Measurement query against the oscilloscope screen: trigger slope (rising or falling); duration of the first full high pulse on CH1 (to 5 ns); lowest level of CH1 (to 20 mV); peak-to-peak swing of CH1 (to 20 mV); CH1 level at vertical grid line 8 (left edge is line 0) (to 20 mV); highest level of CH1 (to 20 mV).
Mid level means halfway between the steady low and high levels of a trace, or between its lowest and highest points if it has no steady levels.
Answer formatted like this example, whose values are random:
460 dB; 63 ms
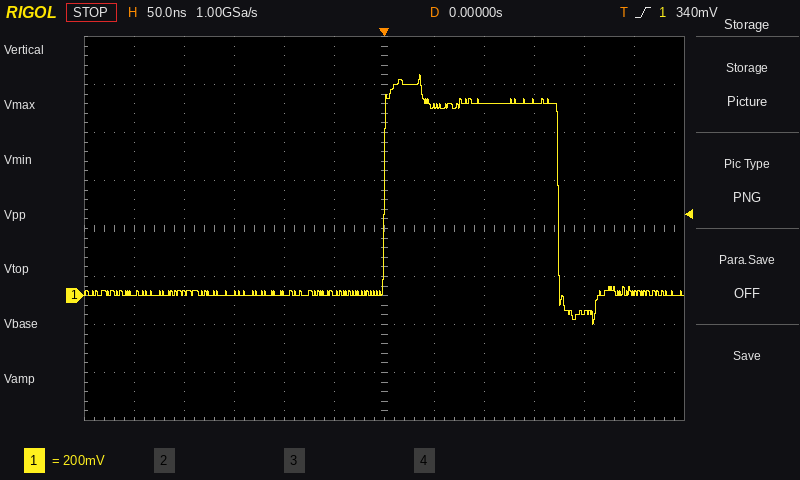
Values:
rising; 175 ns; -120 mV; 1.04 V; 800 mV; 920 mV
